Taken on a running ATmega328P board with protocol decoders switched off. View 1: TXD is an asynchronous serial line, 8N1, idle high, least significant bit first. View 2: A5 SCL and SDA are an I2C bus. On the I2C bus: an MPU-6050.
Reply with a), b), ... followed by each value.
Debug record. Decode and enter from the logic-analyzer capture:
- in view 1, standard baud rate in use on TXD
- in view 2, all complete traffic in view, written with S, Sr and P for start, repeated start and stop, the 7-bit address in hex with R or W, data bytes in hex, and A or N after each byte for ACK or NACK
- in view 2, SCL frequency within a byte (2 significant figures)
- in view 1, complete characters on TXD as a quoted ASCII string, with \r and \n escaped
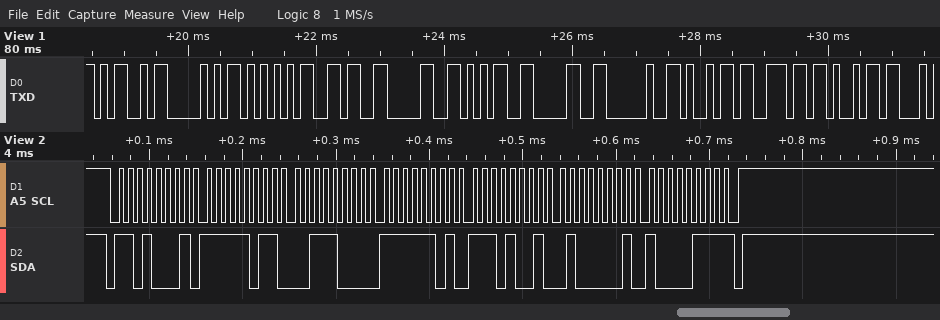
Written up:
a) 9600 baud
b) S 68R A FB A 38 A FD A E9 A 41 A 87 N P
c) 100 kHz
d) "MPU6050 ini"
